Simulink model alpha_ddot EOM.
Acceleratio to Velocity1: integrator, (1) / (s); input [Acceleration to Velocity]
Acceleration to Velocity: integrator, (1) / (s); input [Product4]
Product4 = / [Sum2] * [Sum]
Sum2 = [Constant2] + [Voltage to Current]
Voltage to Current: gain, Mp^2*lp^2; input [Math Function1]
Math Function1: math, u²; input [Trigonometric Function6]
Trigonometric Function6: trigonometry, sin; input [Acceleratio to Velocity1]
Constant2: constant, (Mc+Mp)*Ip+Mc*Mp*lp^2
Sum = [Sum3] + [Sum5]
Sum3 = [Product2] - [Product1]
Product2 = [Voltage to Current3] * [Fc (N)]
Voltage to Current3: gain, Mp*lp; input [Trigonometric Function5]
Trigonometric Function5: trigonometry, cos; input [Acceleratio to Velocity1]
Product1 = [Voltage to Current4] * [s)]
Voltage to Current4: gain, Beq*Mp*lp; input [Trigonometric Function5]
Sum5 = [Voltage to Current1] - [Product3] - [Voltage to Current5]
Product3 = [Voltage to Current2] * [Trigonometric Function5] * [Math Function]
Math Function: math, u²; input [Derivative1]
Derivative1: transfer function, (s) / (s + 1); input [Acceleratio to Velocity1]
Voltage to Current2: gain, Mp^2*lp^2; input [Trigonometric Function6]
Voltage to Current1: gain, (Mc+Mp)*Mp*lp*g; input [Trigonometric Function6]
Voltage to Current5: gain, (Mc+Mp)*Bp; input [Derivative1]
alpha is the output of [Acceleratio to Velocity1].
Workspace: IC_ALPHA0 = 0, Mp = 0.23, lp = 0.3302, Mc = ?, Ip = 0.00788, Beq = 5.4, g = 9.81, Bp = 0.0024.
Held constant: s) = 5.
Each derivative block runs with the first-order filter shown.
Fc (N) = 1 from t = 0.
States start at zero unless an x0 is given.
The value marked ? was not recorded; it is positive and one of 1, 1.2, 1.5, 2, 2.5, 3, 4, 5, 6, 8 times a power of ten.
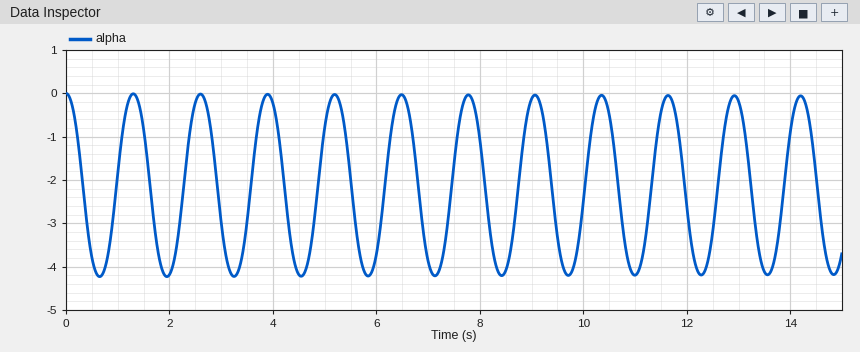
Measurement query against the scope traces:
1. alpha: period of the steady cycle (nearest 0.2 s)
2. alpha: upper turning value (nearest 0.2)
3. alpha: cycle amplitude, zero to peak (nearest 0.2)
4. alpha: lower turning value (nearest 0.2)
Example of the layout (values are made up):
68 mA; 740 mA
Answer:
1.2 s; 0.0; 2.0; -4.2
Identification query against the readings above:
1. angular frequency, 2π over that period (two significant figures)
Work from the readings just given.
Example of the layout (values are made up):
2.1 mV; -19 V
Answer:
5.2 rad/s
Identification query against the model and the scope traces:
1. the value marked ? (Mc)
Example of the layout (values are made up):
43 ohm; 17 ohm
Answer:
1.5
